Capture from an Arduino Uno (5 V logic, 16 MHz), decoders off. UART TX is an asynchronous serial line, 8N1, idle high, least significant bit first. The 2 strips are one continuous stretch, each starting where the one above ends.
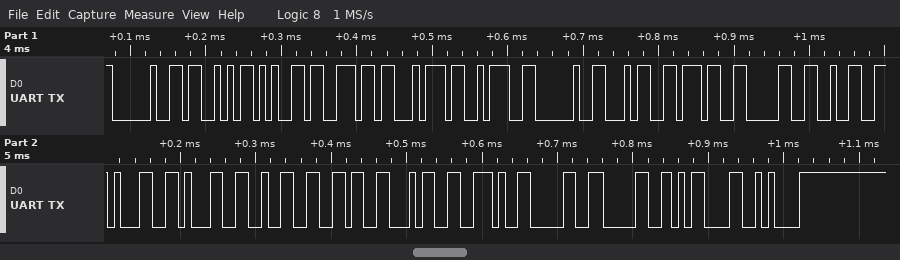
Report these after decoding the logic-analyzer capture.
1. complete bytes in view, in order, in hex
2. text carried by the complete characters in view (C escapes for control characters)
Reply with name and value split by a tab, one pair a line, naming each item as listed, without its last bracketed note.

complete bytes in view, in order, in hex	20 53 65 6E 74 3A 20 34 37 30 32 31 31 32 36 34 2E 30 30 0D 0A
text carried by the complete characters in view	" Sent: 470211264.00\r\n"
